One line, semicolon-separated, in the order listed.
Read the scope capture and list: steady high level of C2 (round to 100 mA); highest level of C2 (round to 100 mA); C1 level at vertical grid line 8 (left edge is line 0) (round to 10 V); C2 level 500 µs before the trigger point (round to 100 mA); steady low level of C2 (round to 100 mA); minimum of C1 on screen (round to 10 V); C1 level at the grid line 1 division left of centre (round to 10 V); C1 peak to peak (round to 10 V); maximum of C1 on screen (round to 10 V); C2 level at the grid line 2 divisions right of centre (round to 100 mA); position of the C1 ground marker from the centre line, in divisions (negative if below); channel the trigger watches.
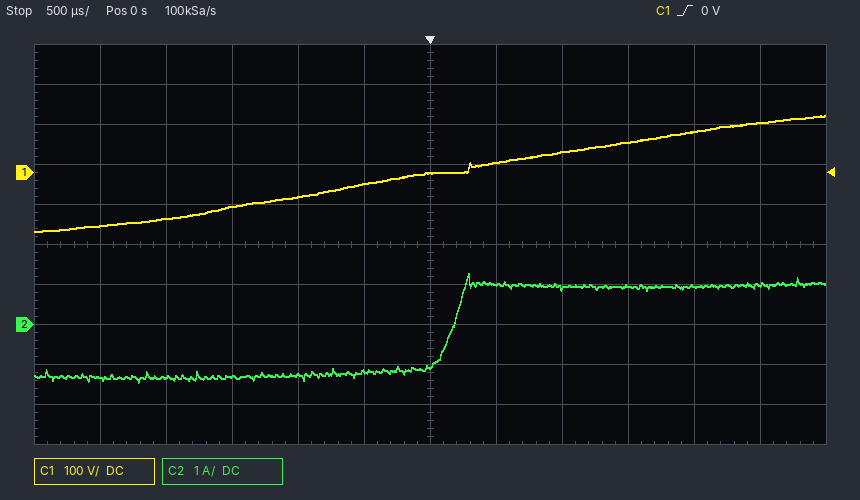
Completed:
1.0 A; 1.3 A; 50 V; -1.2 A; -1.3 A; -150 V; -30 V; 290 V; 140 V; 900 mA; +1.8 div; C1
